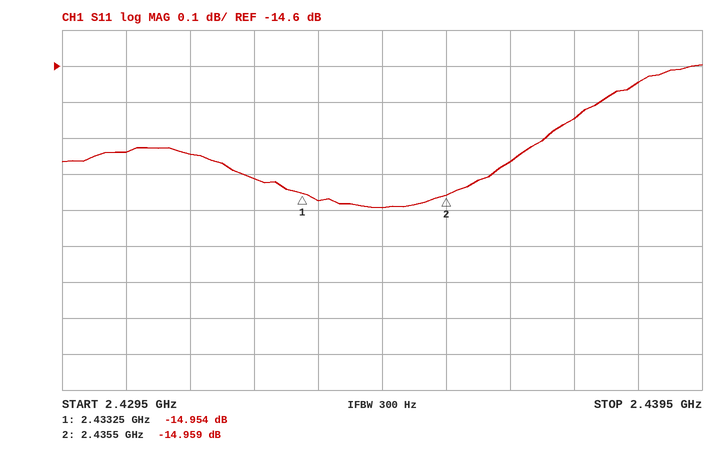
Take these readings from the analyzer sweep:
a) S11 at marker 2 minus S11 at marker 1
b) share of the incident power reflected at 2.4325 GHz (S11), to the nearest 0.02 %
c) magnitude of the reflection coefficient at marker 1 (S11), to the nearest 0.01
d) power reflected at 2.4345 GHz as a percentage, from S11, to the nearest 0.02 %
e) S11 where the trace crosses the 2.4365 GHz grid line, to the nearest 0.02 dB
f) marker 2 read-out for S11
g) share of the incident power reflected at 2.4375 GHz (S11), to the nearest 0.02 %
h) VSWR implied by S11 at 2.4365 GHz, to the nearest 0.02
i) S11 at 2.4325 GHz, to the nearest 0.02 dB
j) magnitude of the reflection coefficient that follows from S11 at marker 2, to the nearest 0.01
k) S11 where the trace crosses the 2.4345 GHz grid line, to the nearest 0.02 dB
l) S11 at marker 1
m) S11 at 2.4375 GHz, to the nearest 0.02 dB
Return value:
-0.005 dB
3.22 %
0.18
3.16 %
-14.86 dB
-14.959 dB
3.36 %
1.44
-14.92 dB
0.18
-15.00 dB
-14.954 dB
-14.74 dB
